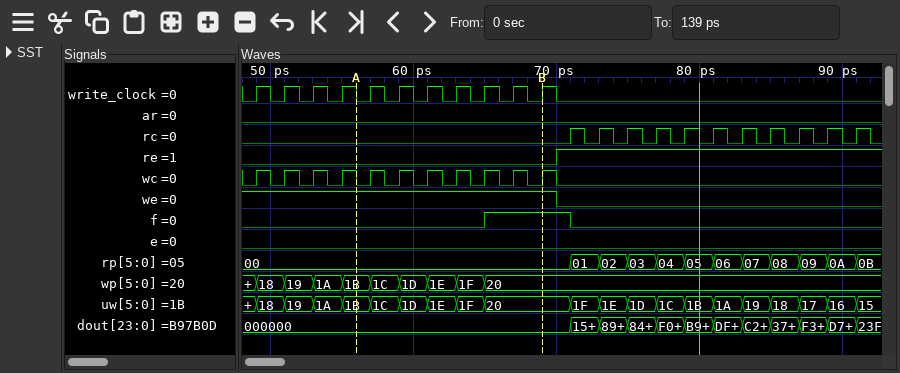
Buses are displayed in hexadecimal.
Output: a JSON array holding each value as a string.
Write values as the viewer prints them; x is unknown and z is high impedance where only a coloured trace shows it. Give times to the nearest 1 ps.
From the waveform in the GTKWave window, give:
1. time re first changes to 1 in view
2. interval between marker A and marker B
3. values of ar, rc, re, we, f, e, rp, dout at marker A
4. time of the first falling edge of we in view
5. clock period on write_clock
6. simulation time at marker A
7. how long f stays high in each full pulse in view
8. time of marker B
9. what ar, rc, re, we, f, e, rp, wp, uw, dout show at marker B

["70 ps", "13 ps", "ar=0, rc=0, re=0, we=1, f=0, e=0, rp=00, dout=000000", "70 ps", "2 ps", "56 ps", "6 ps", "69 ps", "ar=0, rc=0, re=0, we=1, f=1, e=0, rp=00, wp=20, uw=20, dout=000000"]
